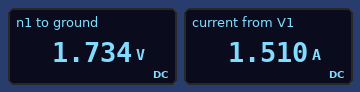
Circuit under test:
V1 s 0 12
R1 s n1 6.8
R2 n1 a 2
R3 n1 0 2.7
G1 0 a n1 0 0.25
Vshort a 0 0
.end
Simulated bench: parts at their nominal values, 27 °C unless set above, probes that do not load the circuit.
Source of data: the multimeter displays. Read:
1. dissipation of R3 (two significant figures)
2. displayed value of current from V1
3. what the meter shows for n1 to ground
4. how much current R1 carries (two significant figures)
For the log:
1.1 W
1.510 A
1.734 V
1.5 A
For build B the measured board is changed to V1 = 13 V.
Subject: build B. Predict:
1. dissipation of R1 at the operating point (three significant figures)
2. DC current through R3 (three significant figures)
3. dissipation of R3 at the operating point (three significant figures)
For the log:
18.2 W
696 mA
1.31 W
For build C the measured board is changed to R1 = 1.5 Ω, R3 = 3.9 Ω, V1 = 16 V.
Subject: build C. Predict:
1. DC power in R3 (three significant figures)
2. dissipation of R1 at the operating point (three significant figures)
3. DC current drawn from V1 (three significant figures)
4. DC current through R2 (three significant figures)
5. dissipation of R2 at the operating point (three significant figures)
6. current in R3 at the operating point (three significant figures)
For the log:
14.4 W
48.2 W
5.67 A
3.75 A
28.1 W
1.92 A
